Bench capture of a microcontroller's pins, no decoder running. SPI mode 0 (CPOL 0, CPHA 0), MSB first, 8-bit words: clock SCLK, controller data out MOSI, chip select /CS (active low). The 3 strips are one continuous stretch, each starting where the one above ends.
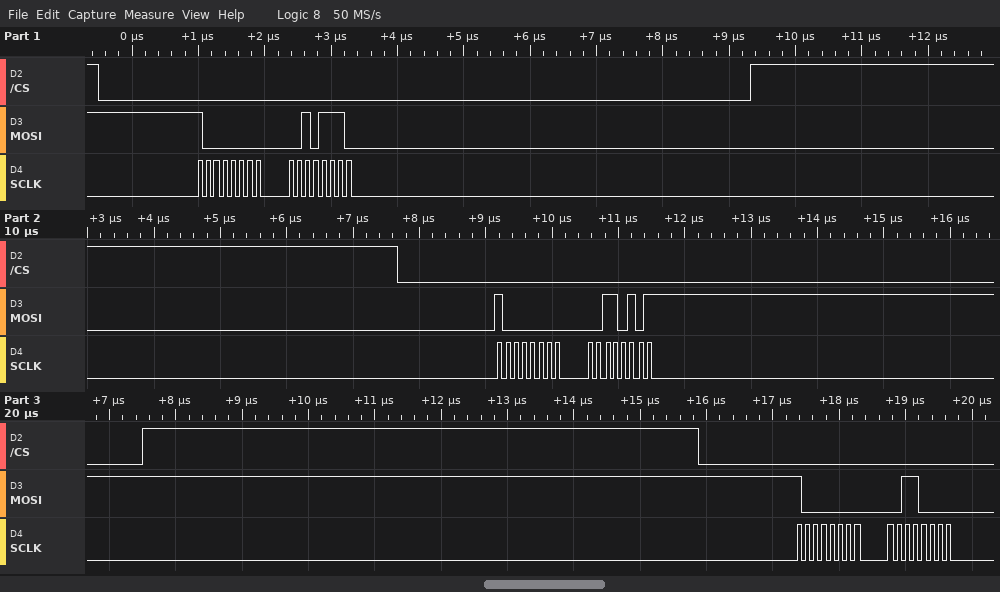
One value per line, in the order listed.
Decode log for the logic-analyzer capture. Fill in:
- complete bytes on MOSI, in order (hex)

80 2E 80 35 80 30
